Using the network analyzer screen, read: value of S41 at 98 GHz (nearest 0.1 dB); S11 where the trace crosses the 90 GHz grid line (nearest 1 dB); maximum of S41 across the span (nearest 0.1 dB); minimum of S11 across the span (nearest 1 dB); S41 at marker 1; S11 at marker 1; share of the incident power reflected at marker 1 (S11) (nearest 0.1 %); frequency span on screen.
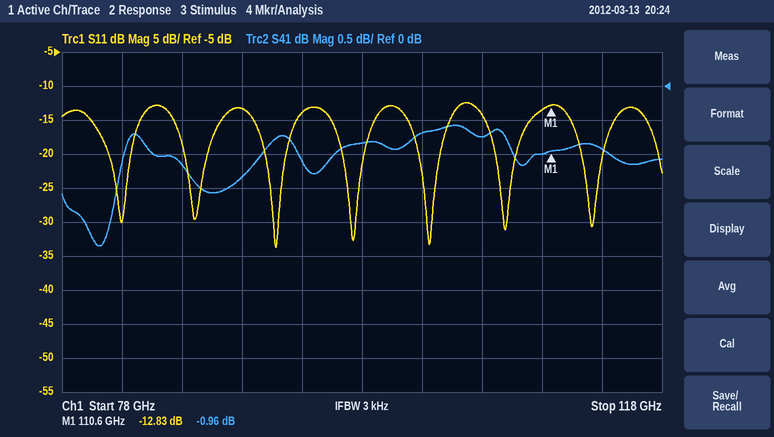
-0.8 dB
-13 dB
-0.6 dB
-34 dB
-0.96 dB
-12.83 dB
5.2 %
40 GHz
